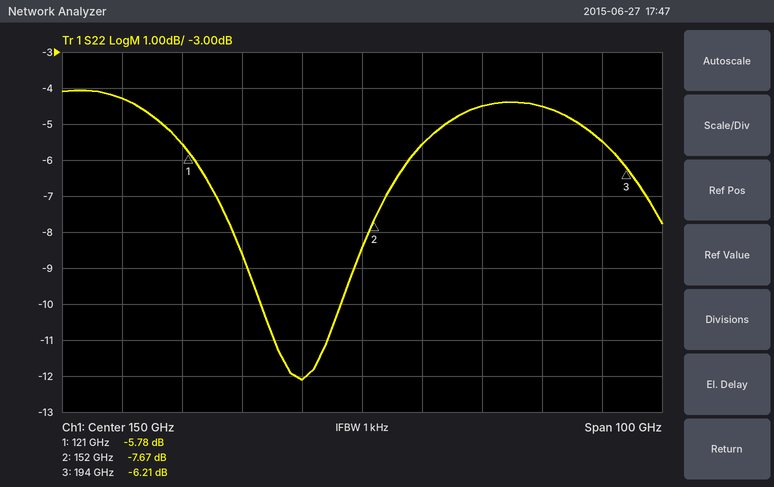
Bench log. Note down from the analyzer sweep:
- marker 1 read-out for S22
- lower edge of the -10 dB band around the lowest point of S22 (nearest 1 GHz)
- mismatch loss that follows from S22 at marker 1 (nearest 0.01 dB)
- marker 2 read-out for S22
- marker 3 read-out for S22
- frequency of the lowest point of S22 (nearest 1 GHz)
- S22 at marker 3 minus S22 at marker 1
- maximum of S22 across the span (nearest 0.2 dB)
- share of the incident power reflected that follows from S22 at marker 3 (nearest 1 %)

-5.78 dB
133 GHz
1.33 dB
-7.67 dB
-6.21 dB
140 GHz
-0.43 dB
-4.0 dB
24 %
